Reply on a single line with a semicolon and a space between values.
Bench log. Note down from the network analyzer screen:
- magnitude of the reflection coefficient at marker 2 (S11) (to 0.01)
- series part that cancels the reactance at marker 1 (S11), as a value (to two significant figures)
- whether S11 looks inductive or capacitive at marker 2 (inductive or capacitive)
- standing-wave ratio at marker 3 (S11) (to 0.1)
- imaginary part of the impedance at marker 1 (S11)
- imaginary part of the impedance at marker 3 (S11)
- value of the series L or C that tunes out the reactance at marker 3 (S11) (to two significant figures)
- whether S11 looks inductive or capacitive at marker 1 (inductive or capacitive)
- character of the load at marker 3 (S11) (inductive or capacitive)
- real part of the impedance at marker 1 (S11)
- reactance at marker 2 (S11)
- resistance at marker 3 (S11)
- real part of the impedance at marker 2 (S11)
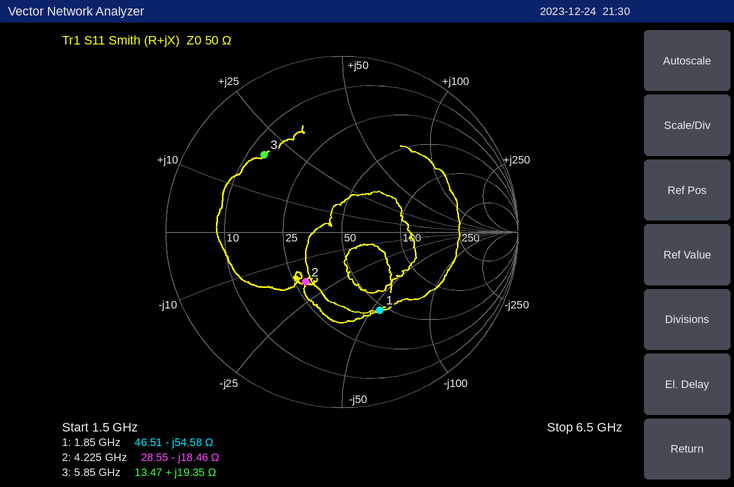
0.35; 4.7 nH; capacitive; 4.3; -54.58 Ω; +19.35 Ω; 1.4 pF; capacitive; inductive; 46.51 Ω; -18.46 Ω; 13.47 Ω; 28.55 Ω
